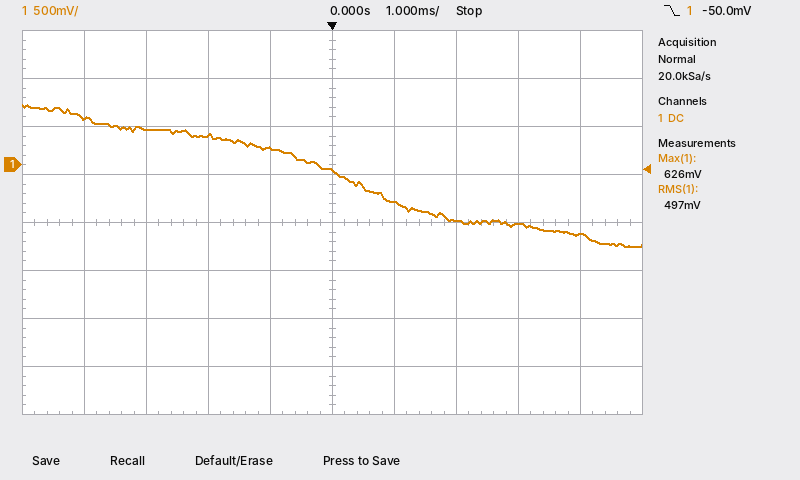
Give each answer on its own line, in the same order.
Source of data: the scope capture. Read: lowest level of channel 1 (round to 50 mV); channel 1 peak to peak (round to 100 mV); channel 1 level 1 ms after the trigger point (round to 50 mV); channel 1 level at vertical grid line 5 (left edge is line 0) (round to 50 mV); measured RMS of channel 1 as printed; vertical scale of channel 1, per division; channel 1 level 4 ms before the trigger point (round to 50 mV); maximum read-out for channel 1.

-850 mV
1.50 V
-400 mV
-50 mV
497 mV
500 mV
500 mV
626 mV
